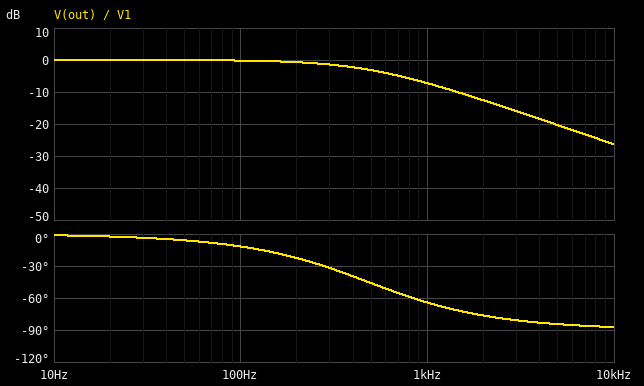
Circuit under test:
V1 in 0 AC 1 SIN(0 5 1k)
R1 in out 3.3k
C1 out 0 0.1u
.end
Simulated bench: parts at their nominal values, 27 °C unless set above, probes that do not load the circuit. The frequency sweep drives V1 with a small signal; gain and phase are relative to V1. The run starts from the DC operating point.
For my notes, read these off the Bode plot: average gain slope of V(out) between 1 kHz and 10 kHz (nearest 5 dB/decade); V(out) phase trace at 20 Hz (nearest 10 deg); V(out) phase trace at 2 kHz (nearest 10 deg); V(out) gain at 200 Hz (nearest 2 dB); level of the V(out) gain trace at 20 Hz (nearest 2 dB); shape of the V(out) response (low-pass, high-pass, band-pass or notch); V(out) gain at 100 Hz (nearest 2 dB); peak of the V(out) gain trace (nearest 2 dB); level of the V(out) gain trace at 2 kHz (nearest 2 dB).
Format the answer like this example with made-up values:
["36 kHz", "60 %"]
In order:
["-20 dB/decade", "0 deg", "-80 deg", "0 dB", "0 dB", "low-pass", "0 dB", "0 dB", "-12 dB"]
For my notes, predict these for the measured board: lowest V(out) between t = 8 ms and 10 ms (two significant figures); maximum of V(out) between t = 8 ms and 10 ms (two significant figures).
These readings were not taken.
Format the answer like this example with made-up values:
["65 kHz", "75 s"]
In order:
["-2.2 V", "2.2 V"]
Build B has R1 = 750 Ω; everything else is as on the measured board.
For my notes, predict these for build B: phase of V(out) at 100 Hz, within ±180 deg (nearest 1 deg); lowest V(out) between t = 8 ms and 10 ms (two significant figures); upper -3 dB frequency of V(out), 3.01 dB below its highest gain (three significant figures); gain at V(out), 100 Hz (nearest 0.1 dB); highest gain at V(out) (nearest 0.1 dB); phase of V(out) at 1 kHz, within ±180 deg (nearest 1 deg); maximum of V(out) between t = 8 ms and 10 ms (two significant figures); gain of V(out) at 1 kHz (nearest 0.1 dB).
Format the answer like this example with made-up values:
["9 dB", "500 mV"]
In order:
["-3 deg", "-4.5 V", "2.12 kHz", "0 dB", "0 dB", "-25 deg", "4.5 V", "-0.9 dB"]
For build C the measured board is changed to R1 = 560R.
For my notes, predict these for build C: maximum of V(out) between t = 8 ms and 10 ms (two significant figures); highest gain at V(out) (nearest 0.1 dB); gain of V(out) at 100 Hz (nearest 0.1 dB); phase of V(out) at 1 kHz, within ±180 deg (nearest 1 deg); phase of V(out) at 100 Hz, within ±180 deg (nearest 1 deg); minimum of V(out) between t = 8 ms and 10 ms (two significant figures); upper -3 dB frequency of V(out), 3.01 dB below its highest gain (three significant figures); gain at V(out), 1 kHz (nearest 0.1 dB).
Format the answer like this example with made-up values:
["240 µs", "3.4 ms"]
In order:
["4.7 V", "0 dB", "0 dB", "-19 deg", "-2 deg", "-4.7 V", "2.84 kHz", "-0.5 dB"]
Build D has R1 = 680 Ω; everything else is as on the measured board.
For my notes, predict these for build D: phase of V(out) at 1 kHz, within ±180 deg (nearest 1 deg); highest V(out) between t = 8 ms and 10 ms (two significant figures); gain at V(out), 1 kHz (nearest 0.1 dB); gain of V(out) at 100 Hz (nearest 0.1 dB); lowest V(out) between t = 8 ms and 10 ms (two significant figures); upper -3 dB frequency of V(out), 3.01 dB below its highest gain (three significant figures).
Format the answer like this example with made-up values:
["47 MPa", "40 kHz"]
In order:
["-23 deg", "4.6 V", "-0.7 dB", "0 dB", "-4.6 V", "2.34 kHz"]
